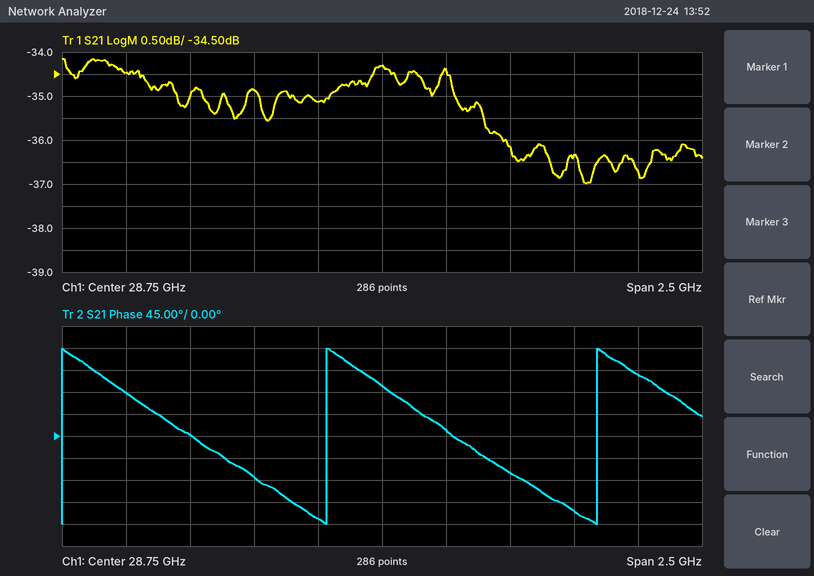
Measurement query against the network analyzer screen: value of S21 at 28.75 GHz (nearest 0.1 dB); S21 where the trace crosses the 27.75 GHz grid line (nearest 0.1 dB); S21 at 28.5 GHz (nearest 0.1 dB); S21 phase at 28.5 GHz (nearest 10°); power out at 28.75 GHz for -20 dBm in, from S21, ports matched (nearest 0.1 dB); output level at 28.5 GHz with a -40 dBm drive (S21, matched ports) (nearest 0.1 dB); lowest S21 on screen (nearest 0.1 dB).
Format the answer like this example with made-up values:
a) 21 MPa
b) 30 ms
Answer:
a) -34.3 dB
b) -34.5 dB
c) -35.1 dB
d) -170°
e) -54.3 dBm
f) -75.1 dBm
g) -37.0 dB
